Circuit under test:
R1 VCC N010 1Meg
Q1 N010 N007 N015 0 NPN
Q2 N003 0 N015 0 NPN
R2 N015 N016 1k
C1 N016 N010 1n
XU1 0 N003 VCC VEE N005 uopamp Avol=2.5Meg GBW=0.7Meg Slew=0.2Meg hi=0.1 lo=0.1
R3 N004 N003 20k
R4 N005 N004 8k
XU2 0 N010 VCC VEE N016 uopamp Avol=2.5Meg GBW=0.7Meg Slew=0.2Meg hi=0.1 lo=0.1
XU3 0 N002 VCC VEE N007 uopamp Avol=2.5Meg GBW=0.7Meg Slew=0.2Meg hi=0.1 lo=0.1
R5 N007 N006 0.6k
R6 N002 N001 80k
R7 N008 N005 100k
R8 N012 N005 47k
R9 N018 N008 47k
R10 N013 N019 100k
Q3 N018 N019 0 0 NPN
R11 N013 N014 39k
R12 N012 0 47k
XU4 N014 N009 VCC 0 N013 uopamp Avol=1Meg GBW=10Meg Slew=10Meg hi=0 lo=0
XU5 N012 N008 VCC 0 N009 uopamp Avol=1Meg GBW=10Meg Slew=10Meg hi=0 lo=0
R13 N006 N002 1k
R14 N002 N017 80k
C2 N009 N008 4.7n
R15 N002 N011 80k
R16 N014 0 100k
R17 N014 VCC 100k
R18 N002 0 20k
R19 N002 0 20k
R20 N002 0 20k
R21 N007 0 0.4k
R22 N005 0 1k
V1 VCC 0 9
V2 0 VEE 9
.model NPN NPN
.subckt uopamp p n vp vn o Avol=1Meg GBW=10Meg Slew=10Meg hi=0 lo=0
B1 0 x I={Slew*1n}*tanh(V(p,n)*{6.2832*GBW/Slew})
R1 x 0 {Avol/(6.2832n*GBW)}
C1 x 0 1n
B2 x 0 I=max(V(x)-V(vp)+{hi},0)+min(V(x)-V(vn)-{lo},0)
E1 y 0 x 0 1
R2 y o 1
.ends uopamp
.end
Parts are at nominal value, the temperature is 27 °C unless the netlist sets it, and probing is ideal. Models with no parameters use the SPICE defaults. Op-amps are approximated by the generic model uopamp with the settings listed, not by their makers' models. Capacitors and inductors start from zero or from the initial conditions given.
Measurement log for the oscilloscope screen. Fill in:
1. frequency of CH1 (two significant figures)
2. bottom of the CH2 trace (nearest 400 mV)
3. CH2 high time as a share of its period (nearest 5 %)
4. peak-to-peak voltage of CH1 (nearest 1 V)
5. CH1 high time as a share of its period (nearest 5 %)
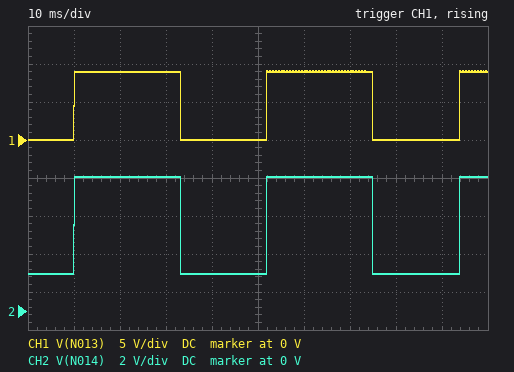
24 Hz
2.0 V
55 %
9 V
55 %
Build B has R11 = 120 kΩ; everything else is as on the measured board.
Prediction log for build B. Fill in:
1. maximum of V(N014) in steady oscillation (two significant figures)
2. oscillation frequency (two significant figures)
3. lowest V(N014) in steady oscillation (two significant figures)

5.8 V
46 Hz
3.2 V
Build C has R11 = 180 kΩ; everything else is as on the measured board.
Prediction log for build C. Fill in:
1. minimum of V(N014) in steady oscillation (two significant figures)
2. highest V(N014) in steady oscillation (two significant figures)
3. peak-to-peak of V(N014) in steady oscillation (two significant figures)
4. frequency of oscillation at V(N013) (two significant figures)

3.5 V
5.5 V
2.0 V
62 Hz
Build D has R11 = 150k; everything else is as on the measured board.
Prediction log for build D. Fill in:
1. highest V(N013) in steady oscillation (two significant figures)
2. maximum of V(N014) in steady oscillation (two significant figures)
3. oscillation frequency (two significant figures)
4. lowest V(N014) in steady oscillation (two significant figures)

9.0 V
5.6 V
54 Hz
3.4 V
